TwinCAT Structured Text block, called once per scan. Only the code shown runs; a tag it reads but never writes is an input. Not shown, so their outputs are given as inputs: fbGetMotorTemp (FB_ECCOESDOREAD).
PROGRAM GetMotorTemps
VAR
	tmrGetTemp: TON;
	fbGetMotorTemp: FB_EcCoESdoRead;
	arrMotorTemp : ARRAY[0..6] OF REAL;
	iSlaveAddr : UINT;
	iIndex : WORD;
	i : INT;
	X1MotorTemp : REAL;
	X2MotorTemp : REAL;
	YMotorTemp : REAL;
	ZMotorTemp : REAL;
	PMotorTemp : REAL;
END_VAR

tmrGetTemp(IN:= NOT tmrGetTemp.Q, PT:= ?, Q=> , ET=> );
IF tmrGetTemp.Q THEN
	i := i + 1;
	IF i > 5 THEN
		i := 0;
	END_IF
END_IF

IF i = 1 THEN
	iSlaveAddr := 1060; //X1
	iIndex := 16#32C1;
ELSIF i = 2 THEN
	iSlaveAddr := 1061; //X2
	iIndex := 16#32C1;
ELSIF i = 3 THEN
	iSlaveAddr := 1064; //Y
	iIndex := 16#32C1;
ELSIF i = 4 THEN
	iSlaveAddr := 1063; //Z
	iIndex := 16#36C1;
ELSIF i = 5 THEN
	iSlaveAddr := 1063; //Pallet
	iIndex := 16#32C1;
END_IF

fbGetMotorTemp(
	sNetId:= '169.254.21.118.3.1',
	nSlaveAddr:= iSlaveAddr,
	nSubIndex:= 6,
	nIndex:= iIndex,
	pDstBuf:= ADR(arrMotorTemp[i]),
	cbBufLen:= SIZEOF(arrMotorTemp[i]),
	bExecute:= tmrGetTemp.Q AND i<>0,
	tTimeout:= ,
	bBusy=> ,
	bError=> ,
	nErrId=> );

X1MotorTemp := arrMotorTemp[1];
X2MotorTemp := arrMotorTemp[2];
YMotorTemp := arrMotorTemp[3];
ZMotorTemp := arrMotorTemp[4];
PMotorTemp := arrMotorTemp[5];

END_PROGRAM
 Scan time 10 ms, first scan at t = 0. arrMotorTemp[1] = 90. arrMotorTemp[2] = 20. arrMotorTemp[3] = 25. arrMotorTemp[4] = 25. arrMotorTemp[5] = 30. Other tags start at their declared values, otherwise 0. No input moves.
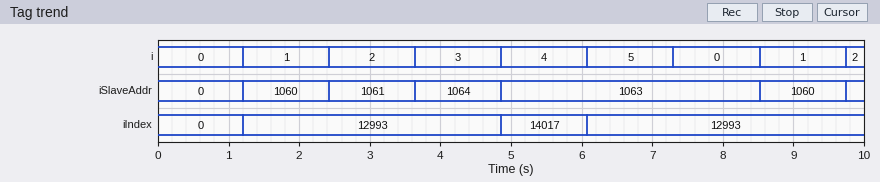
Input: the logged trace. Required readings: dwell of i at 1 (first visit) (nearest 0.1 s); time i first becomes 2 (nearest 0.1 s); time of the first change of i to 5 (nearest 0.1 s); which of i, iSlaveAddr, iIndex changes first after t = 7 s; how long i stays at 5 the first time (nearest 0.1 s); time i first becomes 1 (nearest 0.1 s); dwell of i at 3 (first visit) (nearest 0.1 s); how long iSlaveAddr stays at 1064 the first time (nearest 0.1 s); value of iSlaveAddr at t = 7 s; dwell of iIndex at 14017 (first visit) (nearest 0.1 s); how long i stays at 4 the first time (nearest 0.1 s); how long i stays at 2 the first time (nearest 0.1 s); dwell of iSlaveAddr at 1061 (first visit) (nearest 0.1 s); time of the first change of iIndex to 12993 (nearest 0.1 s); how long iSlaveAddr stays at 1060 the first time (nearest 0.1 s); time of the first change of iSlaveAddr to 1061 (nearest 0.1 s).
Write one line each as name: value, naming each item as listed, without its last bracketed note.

dwell of i at 1 (first visit): 1.2 s
time i first becomes 2: 2.4 s
time of the first change of i to 5: 6.1 s
which of i, iSlaveAddr, iIndex changes first after t = 7 s: i
how long i stays at 5 the first time: 1.2 s
time i first becomes 1: 1.2 s
dwell of i at 3 (first visit): 1.2 s
how long iSlaveAddr stays at 1064 the first time: 1.2 s
value of iSlaveAddr at t = 7 s: 1063
dwell of iIndex at 14017 (first visit): 1.2 s
how long i stays at 4 the first time: 1.2 s
how long i stays at 2 the first time: 1.2 s
dwell of iSlaveAddr at 1061 (first visit): 1.2 s
time of the first change of iIndex to 12993: 1.2 s
how long iSlaveAddr stays at 1060 the first time: 1.2 s
time of the first change of iSlaveAddr to 1061: 2.4 s
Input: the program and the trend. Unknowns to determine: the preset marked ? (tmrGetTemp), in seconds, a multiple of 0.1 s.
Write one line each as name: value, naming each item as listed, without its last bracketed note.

the preset marked ? (tmrGetTemp), in seconds, a multiple of 0.1 s: 1.2 s
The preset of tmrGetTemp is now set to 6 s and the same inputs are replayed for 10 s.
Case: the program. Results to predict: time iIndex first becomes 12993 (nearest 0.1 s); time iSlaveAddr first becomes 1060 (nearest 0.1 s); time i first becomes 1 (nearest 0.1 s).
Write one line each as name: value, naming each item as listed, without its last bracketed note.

time iIndex first becomes 12993: 6.0 s
time iSlaveAddr first becomes 1060: 6.0 s
time i first becomes 1: 6.0 s
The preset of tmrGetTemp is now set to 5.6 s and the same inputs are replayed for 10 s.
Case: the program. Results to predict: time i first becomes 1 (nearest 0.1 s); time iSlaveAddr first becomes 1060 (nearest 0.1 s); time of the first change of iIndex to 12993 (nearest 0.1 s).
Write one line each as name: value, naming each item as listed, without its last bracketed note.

time i first becomes 1: 5.6 s
time iSlaveAddr first becomes 1060: 5.6 s
time of the first change of iIndex to 12993: 5.6 s
